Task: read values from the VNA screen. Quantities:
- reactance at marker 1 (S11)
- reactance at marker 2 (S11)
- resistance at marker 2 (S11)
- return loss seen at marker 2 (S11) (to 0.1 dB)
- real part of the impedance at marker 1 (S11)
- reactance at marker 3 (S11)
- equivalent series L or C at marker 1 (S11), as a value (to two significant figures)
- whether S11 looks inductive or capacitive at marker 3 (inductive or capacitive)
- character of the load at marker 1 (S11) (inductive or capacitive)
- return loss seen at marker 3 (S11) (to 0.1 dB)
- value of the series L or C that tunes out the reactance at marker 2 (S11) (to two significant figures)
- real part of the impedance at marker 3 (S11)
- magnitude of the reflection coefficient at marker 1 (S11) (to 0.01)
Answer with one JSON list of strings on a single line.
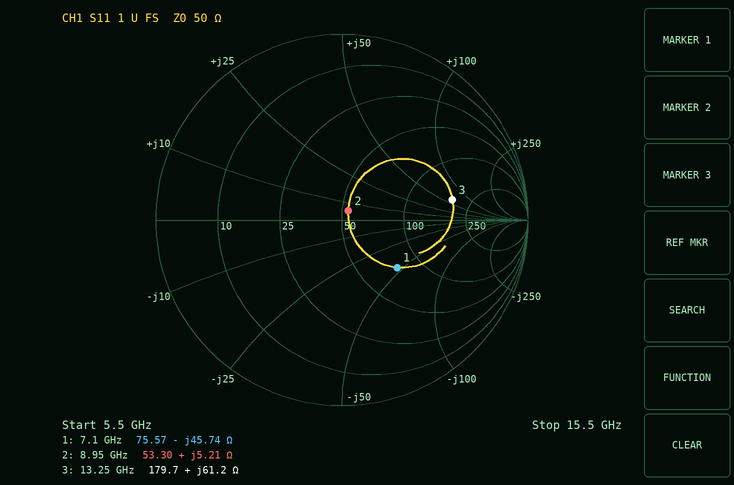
["-45.74 Ω", "+5.21 Ω", "53.30 Ω", "24.5 dB", "75.57 Ω", "+61.2 Ω", "490 fF", "inductive", "capacitive", "4.4 dB", "3.4 pF", "179.7 Ω", "0.39"]
